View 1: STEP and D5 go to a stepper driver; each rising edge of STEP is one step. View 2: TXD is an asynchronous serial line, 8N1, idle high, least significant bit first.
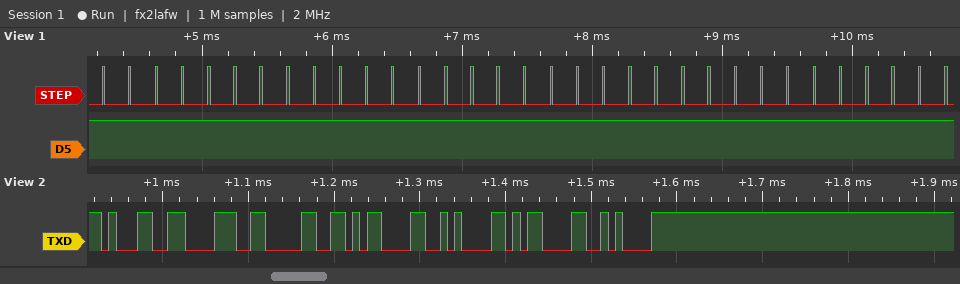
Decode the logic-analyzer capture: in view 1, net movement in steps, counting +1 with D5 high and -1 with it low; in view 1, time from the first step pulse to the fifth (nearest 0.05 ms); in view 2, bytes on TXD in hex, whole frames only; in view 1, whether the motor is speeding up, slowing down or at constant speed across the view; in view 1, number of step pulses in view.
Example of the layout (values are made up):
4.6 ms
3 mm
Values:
+33
0.80 ms
31 38 30 0D 0A 0D 0A
constant speed
33
